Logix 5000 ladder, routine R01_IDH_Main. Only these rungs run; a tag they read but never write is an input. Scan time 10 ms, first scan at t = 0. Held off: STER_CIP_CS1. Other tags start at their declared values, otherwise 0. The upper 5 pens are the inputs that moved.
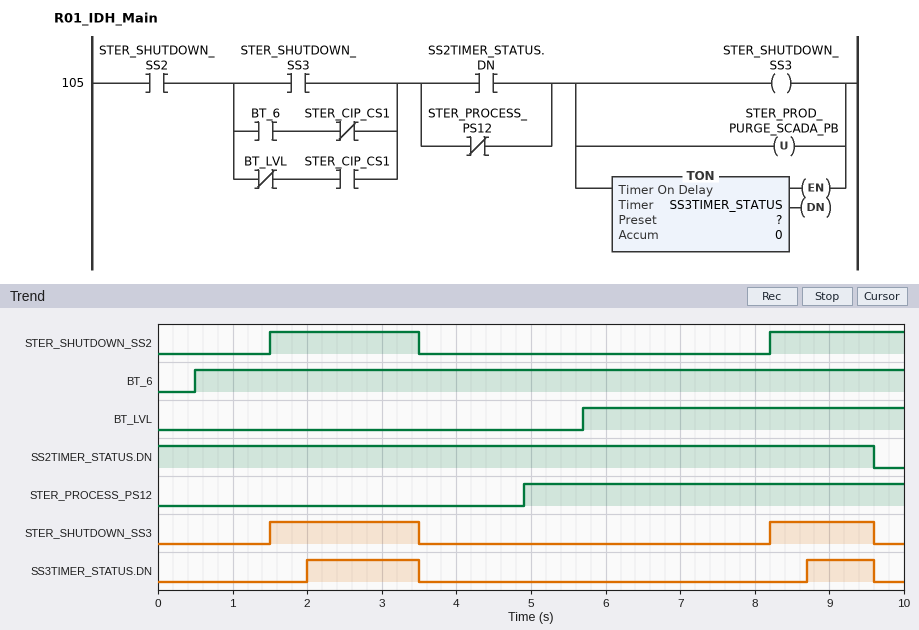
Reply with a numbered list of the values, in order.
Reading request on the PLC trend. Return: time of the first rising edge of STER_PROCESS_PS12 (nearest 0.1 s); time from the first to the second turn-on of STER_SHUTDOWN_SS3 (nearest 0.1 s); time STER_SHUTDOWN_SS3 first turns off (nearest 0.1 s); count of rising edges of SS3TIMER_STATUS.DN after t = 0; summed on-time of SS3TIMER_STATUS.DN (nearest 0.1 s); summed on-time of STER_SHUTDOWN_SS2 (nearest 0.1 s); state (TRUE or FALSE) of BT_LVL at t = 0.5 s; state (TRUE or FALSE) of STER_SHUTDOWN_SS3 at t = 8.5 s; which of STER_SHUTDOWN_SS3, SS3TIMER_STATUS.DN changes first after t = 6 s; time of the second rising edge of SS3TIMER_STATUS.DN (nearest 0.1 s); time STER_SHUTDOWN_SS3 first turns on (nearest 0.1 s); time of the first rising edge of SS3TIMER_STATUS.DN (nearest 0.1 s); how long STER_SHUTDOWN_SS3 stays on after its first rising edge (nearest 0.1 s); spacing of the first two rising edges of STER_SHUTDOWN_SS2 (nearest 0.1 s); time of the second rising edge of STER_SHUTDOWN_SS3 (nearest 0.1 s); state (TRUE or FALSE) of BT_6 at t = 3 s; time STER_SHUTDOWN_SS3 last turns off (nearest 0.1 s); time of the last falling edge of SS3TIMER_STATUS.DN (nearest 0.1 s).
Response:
1. 4.9 s
2. 6.7 s
3. 3.5 s
4. 2
5. 2.4 s
6. 3.8 s
7. FALSE
8. TRUE
9. STER_SHUTDOWN_SS3
10. 8.7 s
11. 1.5 s
12. 2.0 s
13. 2.0 s
14. 6.7 s
15. 8.2 s
16. TRUE
17. 9.6 s
18. 9.6 s
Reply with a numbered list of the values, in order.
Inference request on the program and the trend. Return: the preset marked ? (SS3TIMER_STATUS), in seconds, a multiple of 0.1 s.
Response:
1. 0.5 s
